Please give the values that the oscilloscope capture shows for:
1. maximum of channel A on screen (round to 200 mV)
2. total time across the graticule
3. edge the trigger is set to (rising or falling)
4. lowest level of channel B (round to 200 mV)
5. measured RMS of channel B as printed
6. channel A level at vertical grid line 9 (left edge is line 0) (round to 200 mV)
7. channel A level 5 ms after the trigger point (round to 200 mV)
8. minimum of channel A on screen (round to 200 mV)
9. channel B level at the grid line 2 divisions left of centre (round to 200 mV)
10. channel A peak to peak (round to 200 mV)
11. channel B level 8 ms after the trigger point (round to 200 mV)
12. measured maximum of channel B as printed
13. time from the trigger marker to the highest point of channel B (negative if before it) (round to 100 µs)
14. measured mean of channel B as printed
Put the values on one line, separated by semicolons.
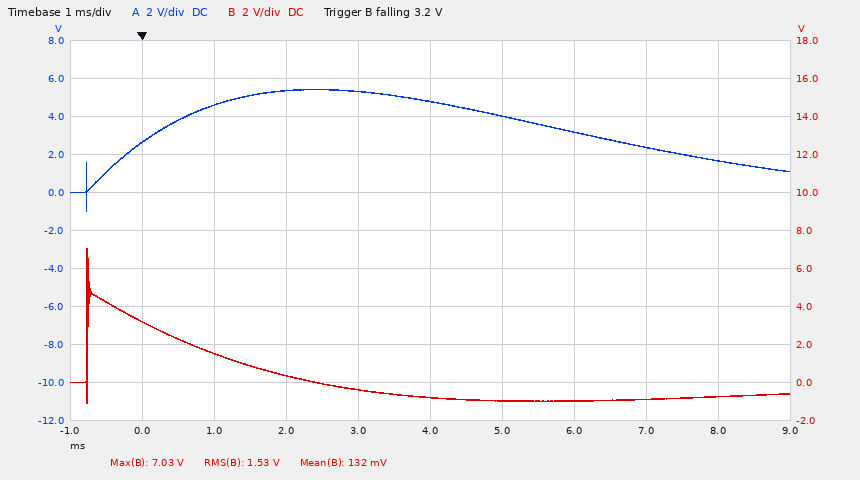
5.4 V; 10 ms; falling; -1.2 V; 1.53 V; 1.6 V; 4.0 V; -1.0 V; 400 mV; 6.4 V; -800 mV; 7.03 V; -800 µs; 132 mV
